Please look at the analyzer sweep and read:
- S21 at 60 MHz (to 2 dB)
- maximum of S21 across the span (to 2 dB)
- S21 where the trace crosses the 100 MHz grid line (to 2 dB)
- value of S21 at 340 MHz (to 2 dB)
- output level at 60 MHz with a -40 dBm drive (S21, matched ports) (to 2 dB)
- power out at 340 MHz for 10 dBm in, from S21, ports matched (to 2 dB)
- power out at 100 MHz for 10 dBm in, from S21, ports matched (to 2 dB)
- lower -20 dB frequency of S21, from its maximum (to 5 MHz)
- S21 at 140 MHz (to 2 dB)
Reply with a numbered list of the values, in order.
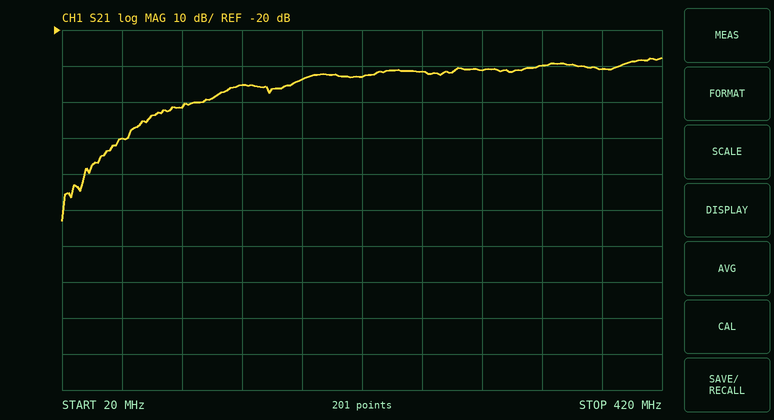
1. -50 dB
2. -28 dB
3. -42 dB
4. -30 dB
5. -90 dBm
6. -20 dBm
7. -32 dBm
8. 65 MHz
9. -36 dB
